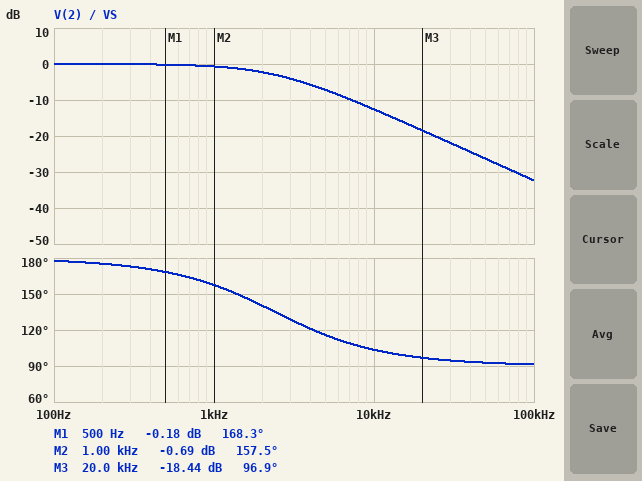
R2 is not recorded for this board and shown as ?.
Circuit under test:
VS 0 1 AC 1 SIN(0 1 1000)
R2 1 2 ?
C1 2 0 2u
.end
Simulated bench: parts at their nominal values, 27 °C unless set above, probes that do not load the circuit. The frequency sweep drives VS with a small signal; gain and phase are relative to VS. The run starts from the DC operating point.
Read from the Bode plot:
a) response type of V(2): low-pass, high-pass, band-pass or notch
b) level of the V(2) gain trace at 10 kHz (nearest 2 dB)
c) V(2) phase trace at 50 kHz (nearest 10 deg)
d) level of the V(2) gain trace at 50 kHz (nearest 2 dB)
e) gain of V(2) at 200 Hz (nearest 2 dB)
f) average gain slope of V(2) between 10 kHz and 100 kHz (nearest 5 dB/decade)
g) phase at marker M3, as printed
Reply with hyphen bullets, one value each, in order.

- low-pass
- -12 dB
- 90 deg
- -26 dB
- 0 dB
- -20 dB/decade
- 96.9 deg
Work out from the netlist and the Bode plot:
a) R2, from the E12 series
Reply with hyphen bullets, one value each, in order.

- 33 Ω
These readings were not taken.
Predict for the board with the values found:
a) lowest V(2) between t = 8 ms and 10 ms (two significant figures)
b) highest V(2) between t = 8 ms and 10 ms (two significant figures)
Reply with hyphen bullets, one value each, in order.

- -920 mV
- 920 mV
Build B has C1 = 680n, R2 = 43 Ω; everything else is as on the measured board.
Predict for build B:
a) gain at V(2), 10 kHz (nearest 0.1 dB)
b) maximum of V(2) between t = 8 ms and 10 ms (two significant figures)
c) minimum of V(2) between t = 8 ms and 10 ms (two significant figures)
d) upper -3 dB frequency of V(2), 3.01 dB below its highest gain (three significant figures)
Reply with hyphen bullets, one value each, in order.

- -6.4 dB
- 980 mV
- -980 mV
- 5.44 kHz
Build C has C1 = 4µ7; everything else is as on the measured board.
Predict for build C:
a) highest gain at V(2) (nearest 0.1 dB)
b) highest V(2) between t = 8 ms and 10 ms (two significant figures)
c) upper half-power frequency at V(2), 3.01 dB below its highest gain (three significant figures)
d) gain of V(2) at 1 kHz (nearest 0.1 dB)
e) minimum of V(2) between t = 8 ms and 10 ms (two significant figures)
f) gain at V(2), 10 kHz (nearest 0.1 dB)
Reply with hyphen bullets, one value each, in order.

- 0 dB
- 720 mV
- 1.03 kHz
- -2.9 dB
- -720 mV
- -19.8 dB
